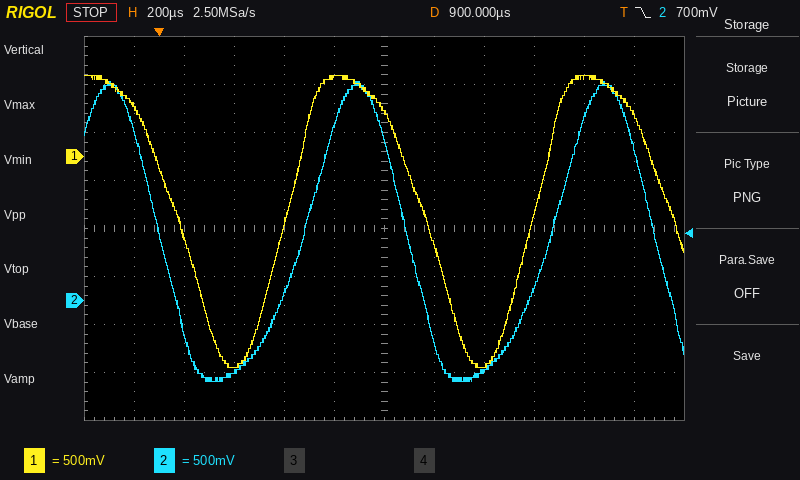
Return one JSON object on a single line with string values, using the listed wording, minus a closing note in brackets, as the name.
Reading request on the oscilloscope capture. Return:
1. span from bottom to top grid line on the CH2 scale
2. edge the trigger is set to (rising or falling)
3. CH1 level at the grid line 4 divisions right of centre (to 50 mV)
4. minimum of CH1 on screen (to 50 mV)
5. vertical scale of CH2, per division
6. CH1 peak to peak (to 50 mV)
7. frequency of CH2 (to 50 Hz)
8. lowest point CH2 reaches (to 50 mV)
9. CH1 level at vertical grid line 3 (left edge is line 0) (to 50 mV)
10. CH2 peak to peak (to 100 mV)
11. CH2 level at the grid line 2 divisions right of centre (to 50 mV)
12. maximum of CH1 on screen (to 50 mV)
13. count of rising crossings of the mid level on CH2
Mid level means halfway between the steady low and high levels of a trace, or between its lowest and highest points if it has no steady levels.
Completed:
{"span from bottom to top grid line on the CH2 scale": "4 V", "edge the trigger is set to": "falling", "CH1 level at the grid line 4 divisions right of centre": "800 mV", "minimum of CH1 on screen": "-2.20 V", "vertical scale of CH2, per division": "500 mV", "CH1 peak to peak": "3.05 V", "frequency of CH2": "1.00 kHz", "lowest point CH2 reaches": "-850 mV", "CH1 level at vertical grid line 3 (left edge is line 0)": "-2.20 V", "CH2 peak to peak": "3.10 V", "CH2 level at the grid line 2 divisions right of centre": "-750 mV", "maximum of CH1 on screen": "850 mV", "count of rising crossings of the mid level on CH2": "2"}
